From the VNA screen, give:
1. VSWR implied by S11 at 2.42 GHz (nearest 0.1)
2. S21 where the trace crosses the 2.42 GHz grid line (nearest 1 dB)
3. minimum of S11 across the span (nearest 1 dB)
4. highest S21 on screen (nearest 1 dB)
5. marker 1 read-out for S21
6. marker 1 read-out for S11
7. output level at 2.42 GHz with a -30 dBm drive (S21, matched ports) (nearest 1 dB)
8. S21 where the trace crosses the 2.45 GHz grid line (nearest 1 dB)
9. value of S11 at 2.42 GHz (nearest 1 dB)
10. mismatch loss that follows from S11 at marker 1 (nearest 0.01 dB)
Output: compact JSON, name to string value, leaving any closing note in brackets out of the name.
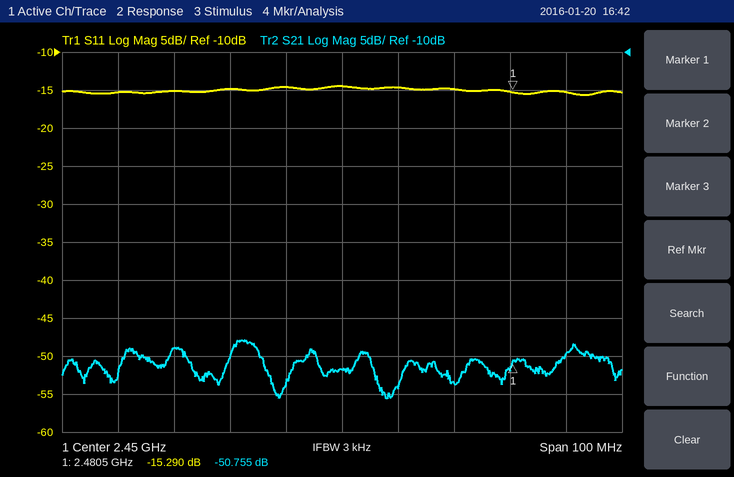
{"VSWR implied by S11 at 2.42 GHz": "1.4", "S21 where the trace crosses the 2.42 GHz grid line": "-49 dB", "minimum of S11 across the span": "-16 dB", "highest S21 on screen": "-48 dB", "marker 1 read-out for S21": "-50.755 dB", "marker 1 read-out for S11": "-15.290 dB", "output level at 2.42 GHz with a -30 dBm drive (S21, matched ports)": "-79 dBm", "S21 where the trace crosses the 2.45 GHz grid line": "-52 dB", "value of S11 at 2.42 GHz": "-15 dB", "mismatch loss that follows from S11 at marker 1": "0.13 dB"}
